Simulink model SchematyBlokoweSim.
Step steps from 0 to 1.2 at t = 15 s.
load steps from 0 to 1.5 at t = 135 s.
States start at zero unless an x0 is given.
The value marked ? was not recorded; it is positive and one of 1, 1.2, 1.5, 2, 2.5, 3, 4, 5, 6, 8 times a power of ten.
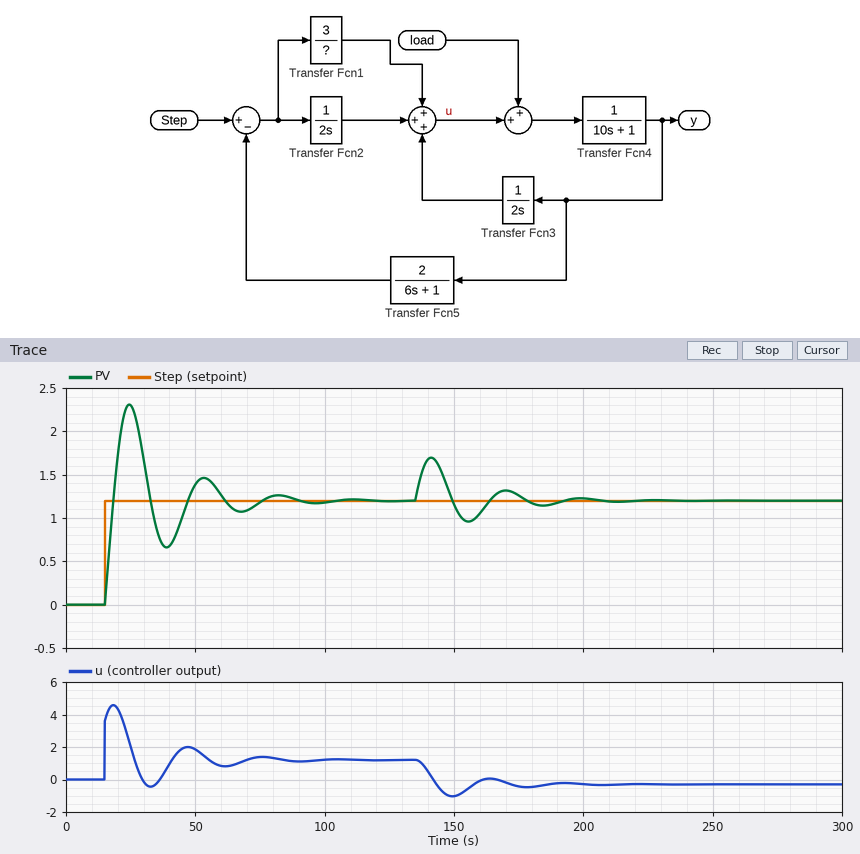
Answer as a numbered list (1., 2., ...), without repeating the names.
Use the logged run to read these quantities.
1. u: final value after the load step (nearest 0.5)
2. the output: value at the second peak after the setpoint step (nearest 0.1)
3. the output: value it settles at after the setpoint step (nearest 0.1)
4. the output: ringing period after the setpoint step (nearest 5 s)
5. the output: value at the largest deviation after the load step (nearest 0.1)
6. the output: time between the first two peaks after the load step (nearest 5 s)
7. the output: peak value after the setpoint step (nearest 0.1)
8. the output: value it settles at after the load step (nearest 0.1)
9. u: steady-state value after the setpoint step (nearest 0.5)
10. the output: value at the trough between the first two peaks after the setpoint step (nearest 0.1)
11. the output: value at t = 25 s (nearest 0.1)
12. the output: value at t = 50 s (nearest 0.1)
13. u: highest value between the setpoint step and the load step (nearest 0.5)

1. -0.5
2. 1.5
3. 1.2
4. 30 s
5. 1.7
6. 30 s
7. 2.3
8. 1.2
9. 1.0
10. 0.7
11. 2.3
12. 1.4
13. 4.5
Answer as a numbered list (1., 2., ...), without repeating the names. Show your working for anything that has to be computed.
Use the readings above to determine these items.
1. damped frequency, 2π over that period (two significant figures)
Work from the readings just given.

1. 2π / 30 = 0.21 rad/s
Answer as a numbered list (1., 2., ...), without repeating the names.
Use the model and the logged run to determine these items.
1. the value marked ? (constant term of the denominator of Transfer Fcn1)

1. 1
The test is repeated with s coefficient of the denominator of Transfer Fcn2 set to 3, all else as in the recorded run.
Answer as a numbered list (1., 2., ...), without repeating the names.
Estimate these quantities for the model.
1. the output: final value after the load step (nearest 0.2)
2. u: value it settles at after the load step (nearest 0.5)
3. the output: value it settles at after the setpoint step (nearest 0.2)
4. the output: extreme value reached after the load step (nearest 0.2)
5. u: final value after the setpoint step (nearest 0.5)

1. 2.4
2. 1.0
3. 2.4
4. 3.0
5. 2.5
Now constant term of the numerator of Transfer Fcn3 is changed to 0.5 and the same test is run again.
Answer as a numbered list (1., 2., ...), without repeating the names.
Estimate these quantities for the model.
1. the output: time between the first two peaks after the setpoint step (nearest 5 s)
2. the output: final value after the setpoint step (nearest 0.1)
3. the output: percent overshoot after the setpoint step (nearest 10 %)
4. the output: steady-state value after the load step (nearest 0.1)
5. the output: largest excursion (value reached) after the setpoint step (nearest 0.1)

1. 25 s
2. 0.8
3. 120 %
4. 0.8
5. 1.8
